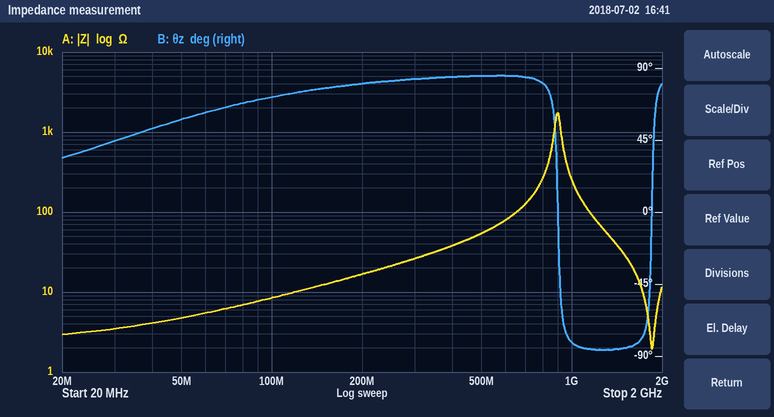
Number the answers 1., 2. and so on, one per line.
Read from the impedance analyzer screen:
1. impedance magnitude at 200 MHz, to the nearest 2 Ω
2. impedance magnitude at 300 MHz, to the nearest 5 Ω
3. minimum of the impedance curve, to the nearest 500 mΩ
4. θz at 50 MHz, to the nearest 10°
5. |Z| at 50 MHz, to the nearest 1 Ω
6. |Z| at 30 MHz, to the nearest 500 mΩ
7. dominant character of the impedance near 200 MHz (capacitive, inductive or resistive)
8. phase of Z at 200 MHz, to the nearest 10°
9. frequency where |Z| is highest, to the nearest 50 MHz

1. 16 Ω
2. 25 Ω
3. 2.0 Ω
4. 60°
5. 5 Ω
6. 3.5 Ω
7. inductive
8. 80°
9. 900 MHz
